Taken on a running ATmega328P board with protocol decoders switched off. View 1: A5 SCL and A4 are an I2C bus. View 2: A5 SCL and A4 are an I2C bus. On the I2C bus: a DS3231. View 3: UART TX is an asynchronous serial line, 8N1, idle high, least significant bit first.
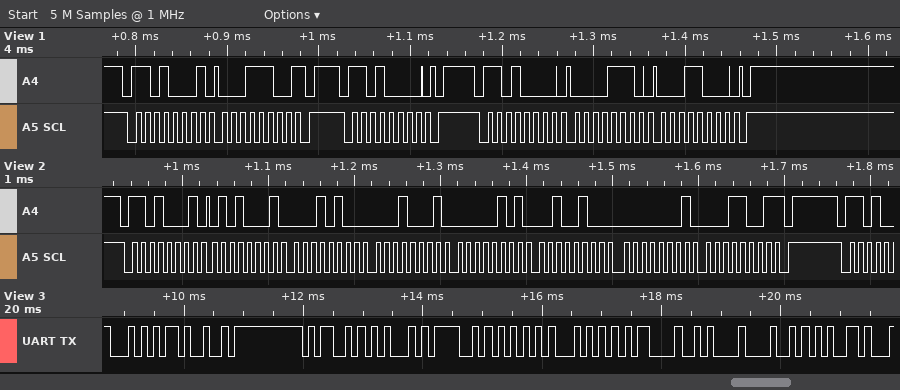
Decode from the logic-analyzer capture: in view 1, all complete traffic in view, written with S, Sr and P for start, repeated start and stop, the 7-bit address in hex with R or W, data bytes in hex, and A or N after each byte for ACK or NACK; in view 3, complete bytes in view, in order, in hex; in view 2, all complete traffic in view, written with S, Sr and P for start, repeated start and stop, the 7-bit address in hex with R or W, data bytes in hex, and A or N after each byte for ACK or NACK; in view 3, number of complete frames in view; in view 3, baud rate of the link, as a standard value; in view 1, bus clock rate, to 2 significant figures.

S 68R A 1C N P S 68W A P S 68W A 0E A 18 A P
54 49 4D 45 4F 55 54 0D 0A 48 65
S 68R A 51 A 14 A 11 A 05 A 24 A 01 A 19 N P
11
9600 baud
100 kHz
